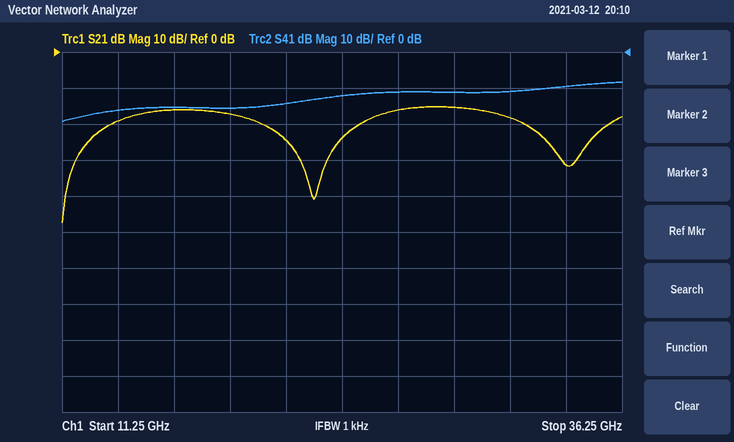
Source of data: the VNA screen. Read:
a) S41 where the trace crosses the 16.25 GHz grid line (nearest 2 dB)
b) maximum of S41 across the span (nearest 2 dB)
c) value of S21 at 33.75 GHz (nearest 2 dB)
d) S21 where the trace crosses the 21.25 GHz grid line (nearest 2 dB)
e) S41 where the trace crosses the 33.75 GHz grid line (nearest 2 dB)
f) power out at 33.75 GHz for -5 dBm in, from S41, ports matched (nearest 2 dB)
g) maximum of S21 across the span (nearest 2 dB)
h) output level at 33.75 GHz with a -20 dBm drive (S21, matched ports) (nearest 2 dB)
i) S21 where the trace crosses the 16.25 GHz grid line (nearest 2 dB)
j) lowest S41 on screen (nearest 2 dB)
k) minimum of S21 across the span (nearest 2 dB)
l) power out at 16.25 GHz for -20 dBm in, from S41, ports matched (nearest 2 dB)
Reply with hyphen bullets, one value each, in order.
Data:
- -16 dB
- -8 dB
- -32 dB
- -24 dB
- -10 dB
- -14 dBm
- -16 dB
- -52 dBm
- -16 dB
- -20 dB
- -48 dB
- -36 dBm
